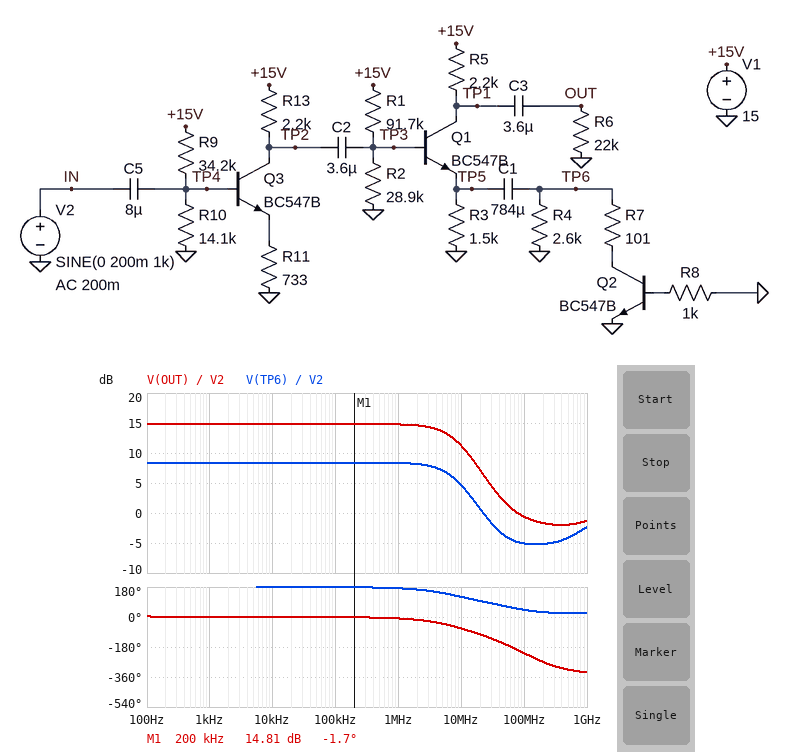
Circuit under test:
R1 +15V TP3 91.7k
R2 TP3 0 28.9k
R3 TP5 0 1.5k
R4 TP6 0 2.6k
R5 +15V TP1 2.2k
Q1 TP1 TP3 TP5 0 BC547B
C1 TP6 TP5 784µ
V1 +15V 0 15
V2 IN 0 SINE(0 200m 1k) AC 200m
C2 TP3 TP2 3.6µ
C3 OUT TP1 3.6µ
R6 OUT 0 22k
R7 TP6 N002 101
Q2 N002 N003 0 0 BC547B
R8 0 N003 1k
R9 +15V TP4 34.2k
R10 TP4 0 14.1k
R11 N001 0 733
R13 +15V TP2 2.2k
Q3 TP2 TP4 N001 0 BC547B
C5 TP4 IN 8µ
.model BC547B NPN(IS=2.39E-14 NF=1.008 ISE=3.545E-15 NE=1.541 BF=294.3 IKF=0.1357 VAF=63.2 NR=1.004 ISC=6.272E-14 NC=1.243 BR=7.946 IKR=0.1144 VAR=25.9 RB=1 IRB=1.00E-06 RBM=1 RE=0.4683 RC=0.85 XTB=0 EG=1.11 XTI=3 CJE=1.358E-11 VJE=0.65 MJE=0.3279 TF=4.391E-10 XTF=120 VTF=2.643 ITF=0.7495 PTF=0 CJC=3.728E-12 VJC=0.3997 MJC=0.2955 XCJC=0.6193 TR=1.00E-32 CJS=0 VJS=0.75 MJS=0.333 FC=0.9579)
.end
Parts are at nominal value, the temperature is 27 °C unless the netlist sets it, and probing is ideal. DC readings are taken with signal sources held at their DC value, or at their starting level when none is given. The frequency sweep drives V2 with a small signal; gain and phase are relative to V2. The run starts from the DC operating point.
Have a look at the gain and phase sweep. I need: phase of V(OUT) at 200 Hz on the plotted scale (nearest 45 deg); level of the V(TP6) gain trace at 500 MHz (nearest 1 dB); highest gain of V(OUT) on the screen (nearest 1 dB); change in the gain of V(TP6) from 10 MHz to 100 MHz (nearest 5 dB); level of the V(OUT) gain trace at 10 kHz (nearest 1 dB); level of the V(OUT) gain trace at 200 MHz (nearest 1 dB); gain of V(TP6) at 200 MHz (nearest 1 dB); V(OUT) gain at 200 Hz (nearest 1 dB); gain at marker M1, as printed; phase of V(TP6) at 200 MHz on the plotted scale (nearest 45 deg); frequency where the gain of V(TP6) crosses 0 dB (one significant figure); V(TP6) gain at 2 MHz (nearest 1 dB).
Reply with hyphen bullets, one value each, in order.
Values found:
- 0 deg
- -4 dB
- 15 dB
- -10 dB
- 15 dB
- -2 dB
- -5 dB
- 15 dB
- 14.81 dB
- 45 deg
- 20 MHz
- 8 dB
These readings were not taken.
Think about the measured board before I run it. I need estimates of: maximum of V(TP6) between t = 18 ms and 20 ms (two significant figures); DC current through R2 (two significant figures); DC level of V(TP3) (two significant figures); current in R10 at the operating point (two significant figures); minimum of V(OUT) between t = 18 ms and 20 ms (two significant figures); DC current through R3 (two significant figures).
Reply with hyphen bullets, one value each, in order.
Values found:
- 530 mV
- 120 µA
- 3.5 V
- 300 µA
- -1.1 V
- 1.9 mA
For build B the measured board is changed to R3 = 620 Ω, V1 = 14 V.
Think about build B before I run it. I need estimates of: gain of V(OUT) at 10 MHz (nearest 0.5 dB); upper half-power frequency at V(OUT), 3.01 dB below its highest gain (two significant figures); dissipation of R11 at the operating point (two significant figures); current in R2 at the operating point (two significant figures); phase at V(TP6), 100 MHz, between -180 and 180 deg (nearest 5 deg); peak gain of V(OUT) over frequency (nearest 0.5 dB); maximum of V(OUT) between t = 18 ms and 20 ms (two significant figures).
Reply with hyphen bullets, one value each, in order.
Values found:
- 13.5 dB
- 5.0 MHz
- 14 mW
- 110 µA
- 55 deg
- 20.5 dB
- 2.1 V
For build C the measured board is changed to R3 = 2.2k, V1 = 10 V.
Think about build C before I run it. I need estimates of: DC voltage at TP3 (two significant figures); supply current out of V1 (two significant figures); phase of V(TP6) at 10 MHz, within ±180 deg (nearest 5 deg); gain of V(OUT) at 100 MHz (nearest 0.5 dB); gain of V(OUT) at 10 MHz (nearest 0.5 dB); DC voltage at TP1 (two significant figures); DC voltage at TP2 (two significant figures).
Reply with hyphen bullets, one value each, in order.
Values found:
- 2.3 V
- 4.0 mA
- 125 deg
- -2.0 dB
- 9.5 dB
- 8.3 V
- 3.6 V
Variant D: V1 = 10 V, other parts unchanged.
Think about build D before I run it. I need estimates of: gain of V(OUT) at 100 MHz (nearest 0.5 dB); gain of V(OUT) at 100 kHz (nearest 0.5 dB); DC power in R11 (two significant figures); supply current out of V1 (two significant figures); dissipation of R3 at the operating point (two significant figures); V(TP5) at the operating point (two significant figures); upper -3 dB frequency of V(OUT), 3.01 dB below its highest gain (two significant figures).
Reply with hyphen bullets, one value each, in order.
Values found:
- -1.5 dB
- 14.5 dB
- 6.3 mW
- 4.3 mA
- 1.9 mW
- 1.7 V
- 8.3 MHz
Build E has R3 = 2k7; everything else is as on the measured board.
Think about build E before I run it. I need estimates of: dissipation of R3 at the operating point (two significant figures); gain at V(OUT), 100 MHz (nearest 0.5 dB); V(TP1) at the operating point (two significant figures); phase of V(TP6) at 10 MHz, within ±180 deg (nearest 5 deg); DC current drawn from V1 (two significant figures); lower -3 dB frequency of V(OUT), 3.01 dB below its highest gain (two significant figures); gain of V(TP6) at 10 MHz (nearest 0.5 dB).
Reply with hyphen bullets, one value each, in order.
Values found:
- 3.1 mW
- -1.5 dB
- 13 V
- 125 deg
- 6.3 mA
- 3.8 Hz
- 5.5 dB
